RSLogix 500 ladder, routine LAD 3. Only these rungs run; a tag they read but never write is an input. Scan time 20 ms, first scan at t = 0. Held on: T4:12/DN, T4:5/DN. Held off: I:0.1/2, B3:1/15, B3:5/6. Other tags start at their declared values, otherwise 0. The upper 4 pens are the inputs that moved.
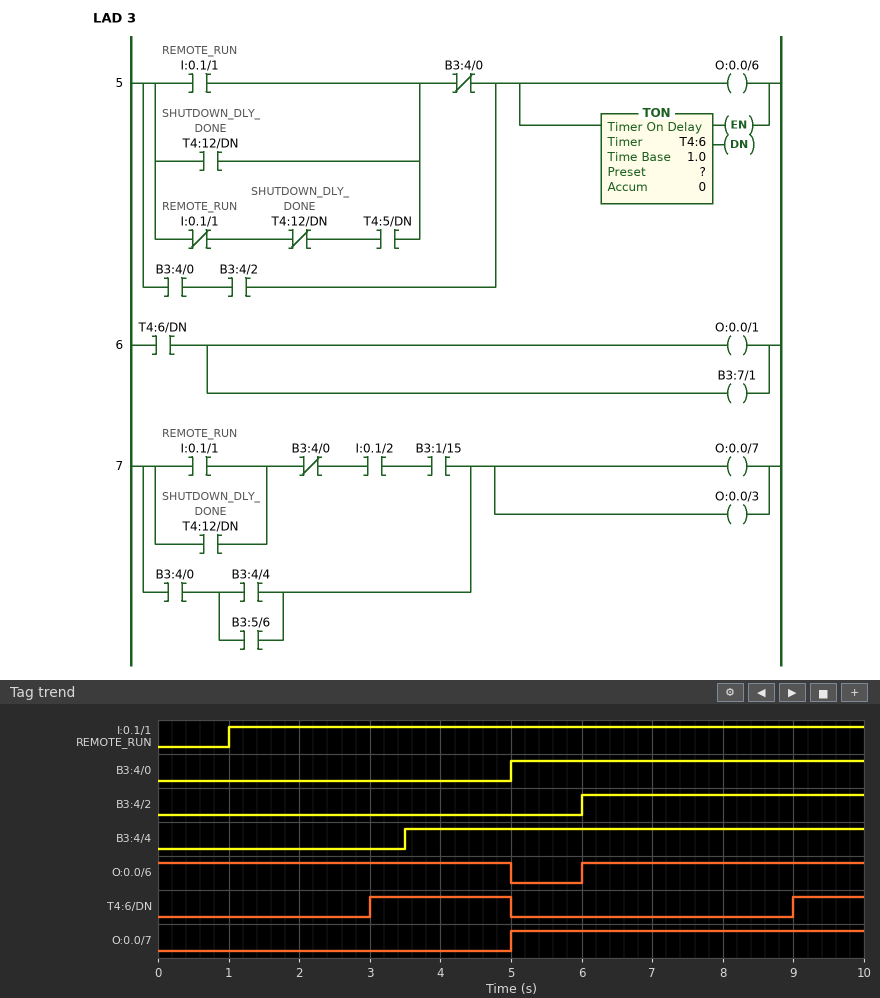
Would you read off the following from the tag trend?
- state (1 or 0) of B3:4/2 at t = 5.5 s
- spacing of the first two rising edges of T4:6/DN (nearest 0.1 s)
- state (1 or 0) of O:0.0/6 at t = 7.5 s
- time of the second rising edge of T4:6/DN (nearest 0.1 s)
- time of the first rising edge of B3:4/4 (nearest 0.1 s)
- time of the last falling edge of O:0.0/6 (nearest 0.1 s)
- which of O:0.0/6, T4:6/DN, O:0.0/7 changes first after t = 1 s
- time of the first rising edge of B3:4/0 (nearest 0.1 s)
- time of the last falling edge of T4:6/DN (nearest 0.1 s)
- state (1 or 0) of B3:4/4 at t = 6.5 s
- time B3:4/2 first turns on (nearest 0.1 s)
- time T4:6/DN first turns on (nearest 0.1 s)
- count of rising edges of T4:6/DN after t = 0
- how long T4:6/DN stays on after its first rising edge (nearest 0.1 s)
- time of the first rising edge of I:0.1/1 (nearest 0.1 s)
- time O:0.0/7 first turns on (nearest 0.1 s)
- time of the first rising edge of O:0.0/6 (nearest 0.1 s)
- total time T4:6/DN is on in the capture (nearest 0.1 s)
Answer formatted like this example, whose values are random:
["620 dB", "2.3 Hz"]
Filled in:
["0", "6.0 s", "1", "9.0 s", "3.5 s", "5.0 s", "T4:6/DN", "5.0 s", "5.0 s", "1", "6.0 s", "3.0 s", "2", "2.0 s", "1.0 s", "5.0 s", "6.0 s", "3.0 s"]
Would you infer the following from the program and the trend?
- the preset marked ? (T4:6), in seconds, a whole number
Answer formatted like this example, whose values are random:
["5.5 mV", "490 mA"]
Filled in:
["3 s"]
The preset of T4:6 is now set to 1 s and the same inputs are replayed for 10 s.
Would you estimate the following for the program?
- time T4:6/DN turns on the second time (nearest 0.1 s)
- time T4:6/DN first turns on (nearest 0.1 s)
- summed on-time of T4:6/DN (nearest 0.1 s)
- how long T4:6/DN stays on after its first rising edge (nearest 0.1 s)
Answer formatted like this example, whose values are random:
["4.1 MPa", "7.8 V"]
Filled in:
["7.0 s", "1.0 s", "7.0 s", "4.0 s"]
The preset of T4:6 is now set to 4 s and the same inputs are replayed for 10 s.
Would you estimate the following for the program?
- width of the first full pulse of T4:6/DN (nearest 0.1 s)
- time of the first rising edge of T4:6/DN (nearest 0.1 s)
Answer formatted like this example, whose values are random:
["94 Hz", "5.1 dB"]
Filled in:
["1.0 s", "4.0 s"]
